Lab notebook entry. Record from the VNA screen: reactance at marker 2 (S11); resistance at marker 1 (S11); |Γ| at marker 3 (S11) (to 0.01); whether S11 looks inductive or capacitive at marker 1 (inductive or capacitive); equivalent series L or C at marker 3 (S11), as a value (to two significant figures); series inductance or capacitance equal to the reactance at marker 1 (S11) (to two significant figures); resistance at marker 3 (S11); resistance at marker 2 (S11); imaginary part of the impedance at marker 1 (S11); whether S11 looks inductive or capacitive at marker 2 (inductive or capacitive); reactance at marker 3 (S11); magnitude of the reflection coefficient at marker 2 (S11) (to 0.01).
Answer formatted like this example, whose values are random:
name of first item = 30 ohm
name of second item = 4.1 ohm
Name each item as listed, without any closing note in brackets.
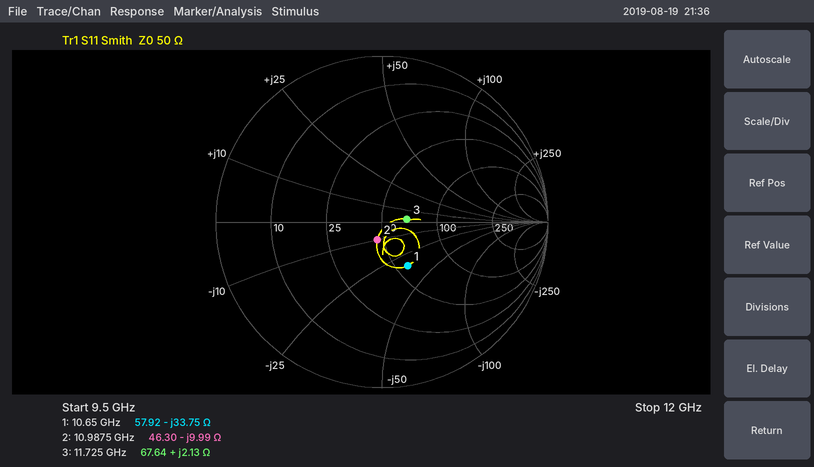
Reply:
reactance at marker 2 = -9.99 Ω
resistance at marker 1 = 57.92 Ω
|Γ| at marker 3 (S11) = 0.15
whether S11 looks inductive or capacitive at marker 1 = capacitive
equivalent series L or C at marker 3 (S11), as a value = 29 pH
series inductance or capacitance equal to the reactance at marker 1 (S11) = 440 fF
resistance at marker 3 = 67.64 Ω
resistance at marker 2 = 46.30 Ω
imaginary part of the impedance at marker 1 = -33.75 Ω
whether S11 looks inductive or capacitive at marker 2 = capacitive
reactance at marker 3 = +2.13 Ω
magnitude of the reflection coefficient at marker 2 (S11) = 0.11
